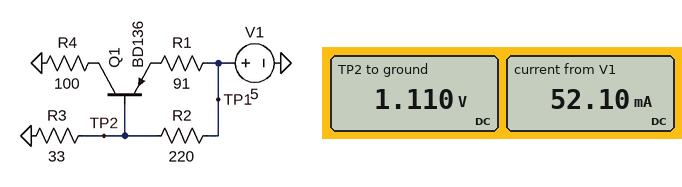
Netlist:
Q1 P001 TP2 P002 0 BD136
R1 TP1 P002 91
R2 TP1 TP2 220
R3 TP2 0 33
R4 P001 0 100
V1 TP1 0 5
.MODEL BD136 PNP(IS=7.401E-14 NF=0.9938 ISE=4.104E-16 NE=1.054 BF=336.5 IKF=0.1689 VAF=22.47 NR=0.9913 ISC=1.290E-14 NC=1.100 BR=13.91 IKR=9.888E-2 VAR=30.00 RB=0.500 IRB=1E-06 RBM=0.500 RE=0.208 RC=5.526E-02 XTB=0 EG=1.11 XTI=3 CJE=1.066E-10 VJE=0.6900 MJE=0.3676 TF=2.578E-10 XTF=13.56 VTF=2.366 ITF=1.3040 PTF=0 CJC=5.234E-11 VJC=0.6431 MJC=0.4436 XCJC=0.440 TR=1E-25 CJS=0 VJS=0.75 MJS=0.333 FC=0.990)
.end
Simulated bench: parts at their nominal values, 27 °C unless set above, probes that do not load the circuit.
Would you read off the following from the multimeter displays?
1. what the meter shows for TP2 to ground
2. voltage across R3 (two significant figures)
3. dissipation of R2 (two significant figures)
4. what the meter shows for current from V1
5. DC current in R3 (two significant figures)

1.110 V
1.1 V
69 mW
52.10 mA
34 mA
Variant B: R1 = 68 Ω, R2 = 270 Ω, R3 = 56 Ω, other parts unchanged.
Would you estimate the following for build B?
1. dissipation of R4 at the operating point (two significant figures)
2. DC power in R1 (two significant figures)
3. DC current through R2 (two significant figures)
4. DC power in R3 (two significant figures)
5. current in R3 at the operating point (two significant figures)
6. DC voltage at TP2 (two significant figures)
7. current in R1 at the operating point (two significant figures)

54 mW
100 mW
13 mA
45 mW
28 mA
1.6 V
39 mA
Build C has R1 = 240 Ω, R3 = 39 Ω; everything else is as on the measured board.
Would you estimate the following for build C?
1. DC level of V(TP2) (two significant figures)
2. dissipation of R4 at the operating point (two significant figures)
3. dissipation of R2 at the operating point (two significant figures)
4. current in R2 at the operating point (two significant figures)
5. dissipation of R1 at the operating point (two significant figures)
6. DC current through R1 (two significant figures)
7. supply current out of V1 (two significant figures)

770 mV
20 mW
81 mW
19 mA
52 mW
15 mA
34 mA
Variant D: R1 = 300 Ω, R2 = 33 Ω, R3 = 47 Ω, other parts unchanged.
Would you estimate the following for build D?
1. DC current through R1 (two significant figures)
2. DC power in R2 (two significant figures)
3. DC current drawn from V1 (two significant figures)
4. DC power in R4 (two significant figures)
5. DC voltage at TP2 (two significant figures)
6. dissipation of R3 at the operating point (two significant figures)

4.7 mA
130 mW
67 mA
2.2 mW
2.9 V
180 mW
